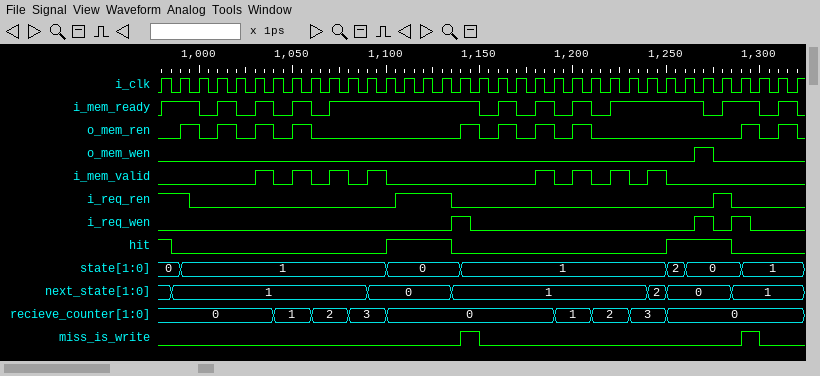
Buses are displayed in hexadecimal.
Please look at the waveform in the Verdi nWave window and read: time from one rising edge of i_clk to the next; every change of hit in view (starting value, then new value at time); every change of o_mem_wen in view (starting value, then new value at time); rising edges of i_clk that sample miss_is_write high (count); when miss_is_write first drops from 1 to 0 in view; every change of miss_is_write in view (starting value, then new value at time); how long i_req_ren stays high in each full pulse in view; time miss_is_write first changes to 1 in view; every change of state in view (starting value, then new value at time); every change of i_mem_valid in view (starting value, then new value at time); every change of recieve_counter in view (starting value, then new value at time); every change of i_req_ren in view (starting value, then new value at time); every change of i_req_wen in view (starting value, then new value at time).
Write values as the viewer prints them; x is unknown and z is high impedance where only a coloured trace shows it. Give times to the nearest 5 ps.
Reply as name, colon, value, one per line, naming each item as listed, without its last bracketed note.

time from one rising edge of i_clk to the next: 10 ps
every change of hit in view: 1, 0 at 985 ps, 1 at 1100 ps, 0 at 1135 ps, 1 at 1250 ps, 0 at 1285 ps
every change of o_mem_wen in view: 0, 1 at 1265 ps, 0 at 1275 ps
rising edges of i_clk that sample miss_is_write high: 2
when miss_is_write first drops from 1 to 0 in view: 1150 ps
every change of miss_is_write in view: 0, 1 at 1140 ps, 0 at 1150 ps, 1 at 1290 ps, 0 at 1300 ps
how long i_req_ren stays high in each full pulse in view: 30 ps, 10 ps
time miss_is_write first changes to 1 in view: 1140 ps
every change of state in view: 0, 1 at 990 ps, 0 at 1100 ps, 1 at 1140 ps, 2 at 1250 ps, 0 at 1260 ps, 1 at 1290 ps
every change of i_mem_valid in view: 0, 1 at 1030 ps, 0 at 1040 ps, 1 at 1050 ps, 0 at 1060 ps, 1 at 1070 ps, 0 at 1080 ps, 1 at 1090 ps, 0 at 1100 ps, 1 at 1180 ps, 0 at 1190 ps, 1 at 1200 ps, 0 at 1210 ps, 1 at 1220 ps, 0 at 1230 ps, 1 at 1240 ps, 0 at 1250 ps
every change of recieve_counter in view: 0, 1 at 1040 ps, 2 at 1060 ps, 3 at 1080 ps, 0 at 1100 ps, 1 at 1190 ps, 2 at 1210 ps, 3 at 1230 ps, 0 at 1250 ps
every change of i_req_ren in view: 1, 0 at 995 ps, 1 at 1105 ps, 0 at 1135 ps, 1 at 1275 ps, 0 at 1285 ps
every change of i_req_wen in view: 0, 1 at 1135 ps, 0 at 1145 ps, 1 at 1265 ps, 0 at 1275 ps, 1 at 1285 ps, 0 at 1295 ps
